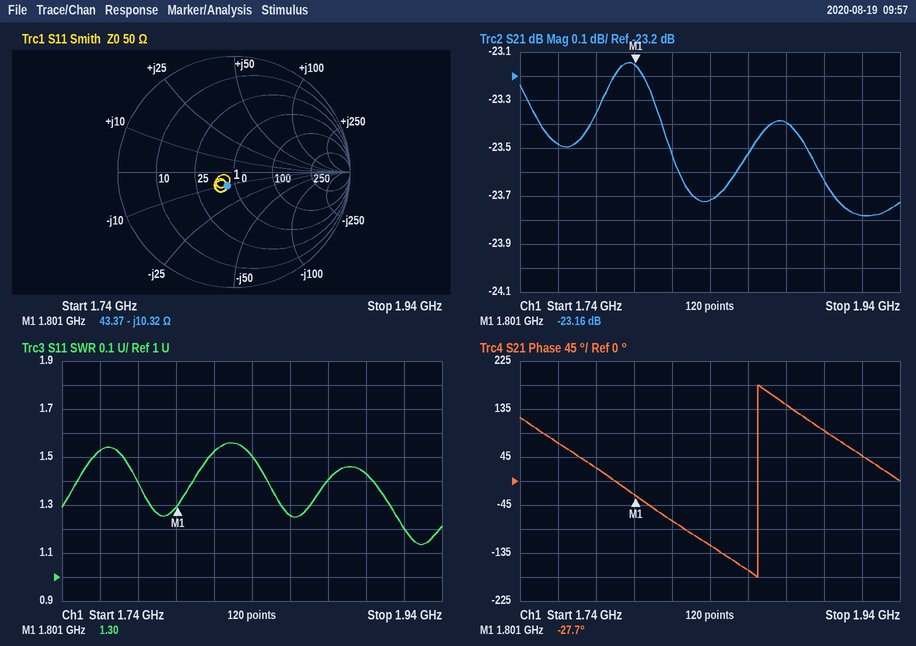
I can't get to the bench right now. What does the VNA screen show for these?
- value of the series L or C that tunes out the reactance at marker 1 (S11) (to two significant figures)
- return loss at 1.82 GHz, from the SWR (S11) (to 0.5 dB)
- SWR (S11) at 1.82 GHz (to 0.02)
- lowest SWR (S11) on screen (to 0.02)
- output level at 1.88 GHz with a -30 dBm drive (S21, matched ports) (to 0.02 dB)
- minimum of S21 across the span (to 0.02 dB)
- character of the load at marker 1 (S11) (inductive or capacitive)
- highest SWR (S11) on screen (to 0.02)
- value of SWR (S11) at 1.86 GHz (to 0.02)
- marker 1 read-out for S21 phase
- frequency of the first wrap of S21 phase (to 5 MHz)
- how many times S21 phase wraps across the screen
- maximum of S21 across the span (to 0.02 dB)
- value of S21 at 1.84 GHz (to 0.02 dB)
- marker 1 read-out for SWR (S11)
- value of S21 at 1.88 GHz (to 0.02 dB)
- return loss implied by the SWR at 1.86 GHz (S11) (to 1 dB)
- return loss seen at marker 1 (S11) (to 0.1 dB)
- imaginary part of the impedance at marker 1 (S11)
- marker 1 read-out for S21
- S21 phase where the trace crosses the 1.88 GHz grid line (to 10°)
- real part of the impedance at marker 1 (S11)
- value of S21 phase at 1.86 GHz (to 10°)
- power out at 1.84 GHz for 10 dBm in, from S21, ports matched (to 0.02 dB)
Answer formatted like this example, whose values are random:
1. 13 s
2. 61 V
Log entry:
1. 910 pH
2. 13.5 dB
3. 1.52
4. 1.14
5. -53.40 dBm
6. -23.78 dB
7. capacitive
8. 1.56
9. 1.26
10. -27.7°
11. 1.865 GHz
12. 1
13. -23.14 dB
14. -23.72 dB
15. 1.30
16. -23.40 dB
17. 19 dB
18. 17.7 dB
19. -10.32 Ω
20. -23.16 dB
21. 140°
22. 43.37 Ω
23. -170°
24. -13.72 dBm
